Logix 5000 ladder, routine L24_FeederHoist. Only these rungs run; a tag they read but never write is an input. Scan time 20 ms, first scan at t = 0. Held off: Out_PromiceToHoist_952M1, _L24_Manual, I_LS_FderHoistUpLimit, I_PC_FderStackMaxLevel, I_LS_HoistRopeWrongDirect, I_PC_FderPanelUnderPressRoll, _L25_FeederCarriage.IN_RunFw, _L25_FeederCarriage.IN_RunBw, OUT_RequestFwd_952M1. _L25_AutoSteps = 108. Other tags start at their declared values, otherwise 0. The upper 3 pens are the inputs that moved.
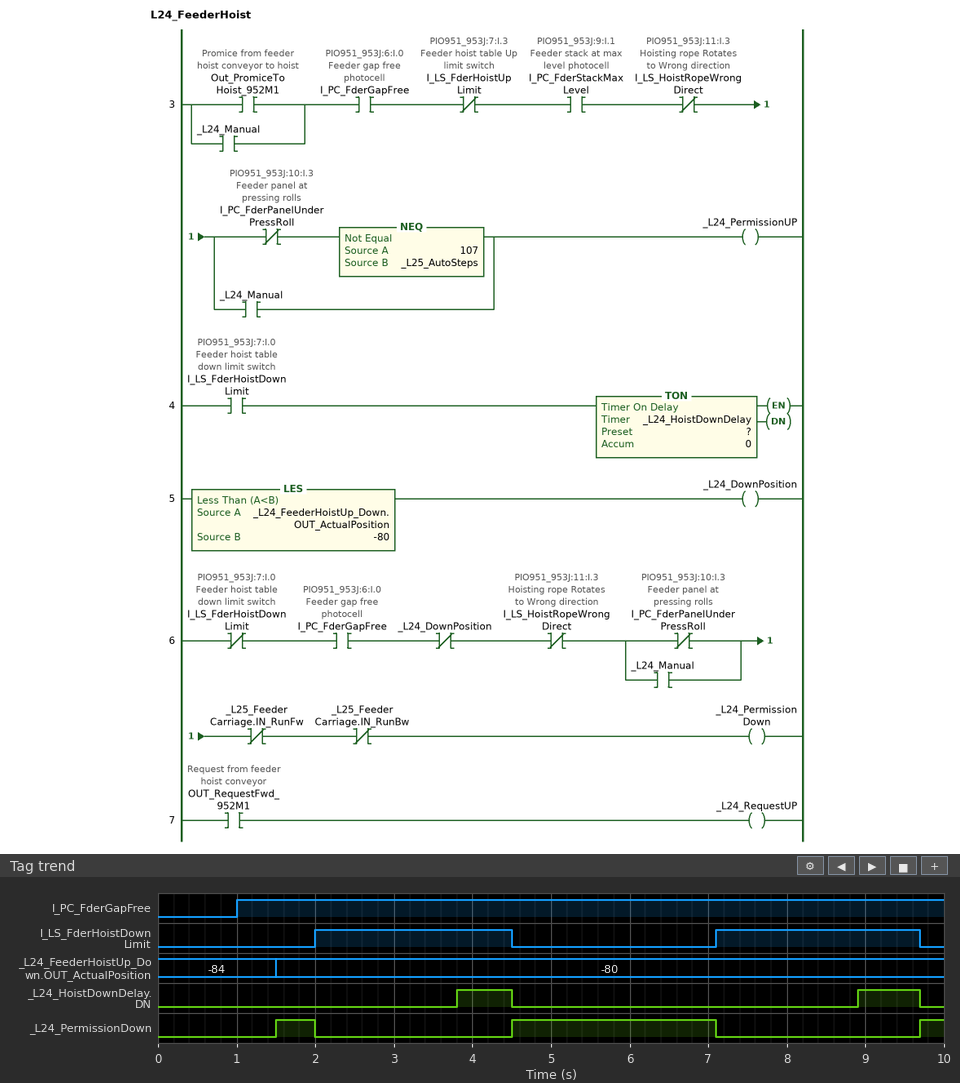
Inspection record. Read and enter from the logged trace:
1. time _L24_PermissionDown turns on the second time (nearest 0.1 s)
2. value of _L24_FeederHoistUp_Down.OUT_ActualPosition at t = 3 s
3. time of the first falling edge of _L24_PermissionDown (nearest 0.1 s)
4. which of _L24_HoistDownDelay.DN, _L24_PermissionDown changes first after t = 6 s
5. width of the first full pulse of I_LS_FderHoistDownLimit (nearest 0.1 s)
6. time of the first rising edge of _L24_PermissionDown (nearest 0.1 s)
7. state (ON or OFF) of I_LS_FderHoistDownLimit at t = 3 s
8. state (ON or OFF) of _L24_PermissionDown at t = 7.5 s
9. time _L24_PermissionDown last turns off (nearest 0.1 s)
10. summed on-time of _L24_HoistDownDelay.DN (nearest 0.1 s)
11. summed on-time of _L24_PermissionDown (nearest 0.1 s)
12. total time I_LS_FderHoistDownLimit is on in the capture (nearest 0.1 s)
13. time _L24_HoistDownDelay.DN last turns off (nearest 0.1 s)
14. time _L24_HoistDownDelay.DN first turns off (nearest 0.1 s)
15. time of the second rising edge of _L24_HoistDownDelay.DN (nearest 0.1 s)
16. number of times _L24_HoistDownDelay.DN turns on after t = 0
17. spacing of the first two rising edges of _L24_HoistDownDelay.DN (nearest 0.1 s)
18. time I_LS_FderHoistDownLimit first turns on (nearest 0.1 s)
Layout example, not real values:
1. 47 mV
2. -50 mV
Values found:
1. 4.5 s
2. -80
3. 2.0 s
4. _L24_PermissionDown
5. 2.5 s
6. 1.5 s
7. ON
8. OFF
9. 7.1 s
10. 1.5 s
11. 3.4 s
12. 5.1 s
13. 9.7 s
14. 4.5 s
15. 8.9 s
16. 2
17. 5.1 s
18. 2.0 s
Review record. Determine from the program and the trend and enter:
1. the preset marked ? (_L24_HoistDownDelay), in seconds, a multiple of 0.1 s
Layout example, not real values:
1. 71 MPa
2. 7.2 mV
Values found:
1. 1.8 s
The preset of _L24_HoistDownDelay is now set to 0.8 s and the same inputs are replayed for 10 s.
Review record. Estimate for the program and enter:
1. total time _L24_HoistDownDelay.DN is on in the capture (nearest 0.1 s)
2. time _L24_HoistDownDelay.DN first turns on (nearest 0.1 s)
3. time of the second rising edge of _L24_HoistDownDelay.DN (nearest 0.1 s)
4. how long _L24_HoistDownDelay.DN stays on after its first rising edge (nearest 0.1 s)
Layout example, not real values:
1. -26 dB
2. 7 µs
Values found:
1. 3.5 s
2. 2.8 s
3. 7.9 s
4. 1.7 s
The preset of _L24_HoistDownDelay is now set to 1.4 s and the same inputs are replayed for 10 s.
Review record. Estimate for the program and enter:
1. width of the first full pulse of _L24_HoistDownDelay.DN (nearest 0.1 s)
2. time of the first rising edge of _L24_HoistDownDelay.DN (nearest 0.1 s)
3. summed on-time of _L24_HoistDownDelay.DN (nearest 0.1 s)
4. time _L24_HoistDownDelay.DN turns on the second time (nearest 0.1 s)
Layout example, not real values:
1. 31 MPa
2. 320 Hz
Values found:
1. 1.1 s
2. 3.4 s
3. 2.3 s
4. 8.5 s
